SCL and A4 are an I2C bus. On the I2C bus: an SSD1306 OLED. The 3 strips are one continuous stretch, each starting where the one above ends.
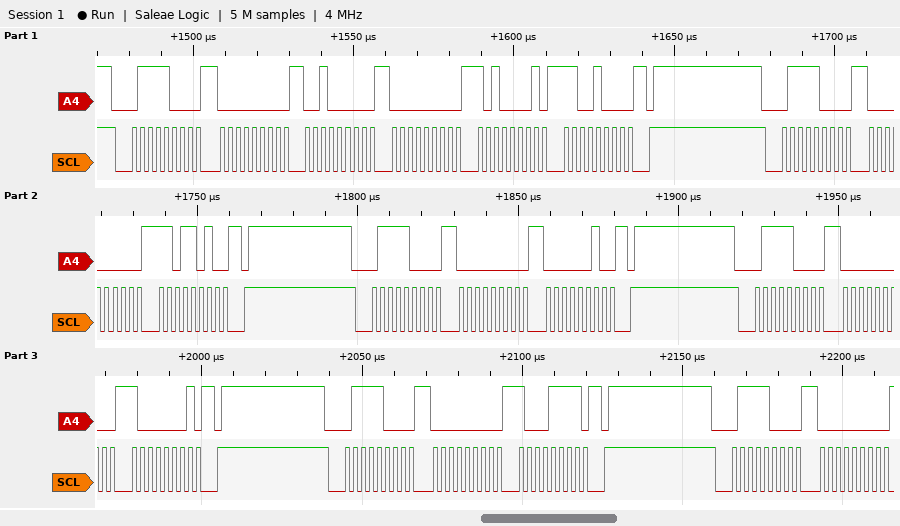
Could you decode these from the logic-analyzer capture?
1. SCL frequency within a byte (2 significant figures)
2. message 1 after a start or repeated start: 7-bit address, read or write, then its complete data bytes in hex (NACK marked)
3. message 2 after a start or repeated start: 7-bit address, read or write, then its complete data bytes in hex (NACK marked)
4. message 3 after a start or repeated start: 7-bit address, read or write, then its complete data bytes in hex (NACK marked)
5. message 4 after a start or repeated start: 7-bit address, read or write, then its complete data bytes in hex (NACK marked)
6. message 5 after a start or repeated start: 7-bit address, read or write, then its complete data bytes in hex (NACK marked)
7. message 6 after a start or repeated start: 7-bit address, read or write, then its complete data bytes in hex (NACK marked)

400 kHz
0x3C write: 00 20 00 A1 C8
0x3C write: 00 DA
0x3C write: 00 02
0x3C write: 00 81
0x3C write: 00 8F
0x3C write: 00
